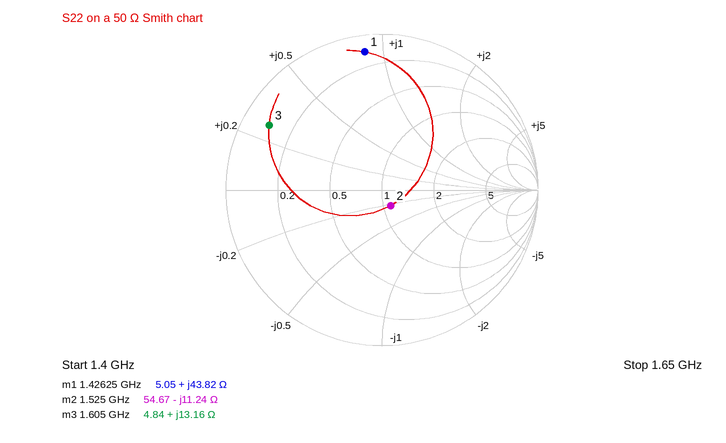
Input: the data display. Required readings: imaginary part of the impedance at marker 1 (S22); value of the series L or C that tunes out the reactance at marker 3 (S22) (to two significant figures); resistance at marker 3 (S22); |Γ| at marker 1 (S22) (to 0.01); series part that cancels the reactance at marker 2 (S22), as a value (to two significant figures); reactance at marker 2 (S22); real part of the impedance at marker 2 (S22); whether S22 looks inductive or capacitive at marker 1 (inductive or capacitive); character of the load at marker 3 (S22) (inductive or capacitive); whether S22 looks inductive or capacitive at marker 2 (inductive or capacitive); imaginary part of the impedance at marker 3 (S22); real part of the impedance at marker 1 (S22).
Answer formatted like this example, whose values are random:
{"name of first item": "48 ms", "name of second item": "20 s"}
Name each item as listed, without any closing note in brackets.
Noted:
{"imaginary part of the impedance at marker 1": "+43.82 Ω", "value of the series L or C that tunes out the reactance at marker 3 (S22)": "7.5 pF", "resistance at marker 3": "4.84 Ω", "|Γ| at marker 1 (S22)": "0.89", "series part that cancels the reactance at marker 2 (S22), as a value": "1.2 nH", "reactance at marker 2": "-11.24 Ω", "real part of the impedance at marker 2": "54.67 Ω", "whether S22 looks inductive or capacitive at marker 1": "inductive", "character of the load at marker 3 (S22)": "inductive", "whether S22 looks inductive or capacitive at marker 2": "capacitive", "imaginary part of the impedance at marker 3": "+13.16 Ω", "real part of the impedance at marker 1": "5.05 Ω"}
